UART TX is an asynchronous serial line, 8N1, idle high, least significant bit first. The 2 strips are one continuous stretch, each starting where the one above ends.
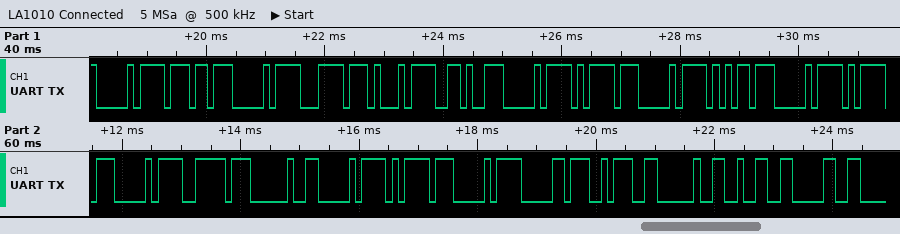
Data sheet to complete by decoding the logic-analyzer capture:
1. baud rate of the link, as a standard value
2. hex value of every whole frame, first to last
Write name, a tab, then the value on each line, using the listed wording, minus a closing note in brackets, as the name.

baud rate of the link, as a standard value	9600 baud
hex value of every whole frame, first to last	D0 B7 D0 BC D1 96 D0 BD D0 B5 D0 BD D0 BE 20 D0 BD D0 B0 3A 20 32 30
